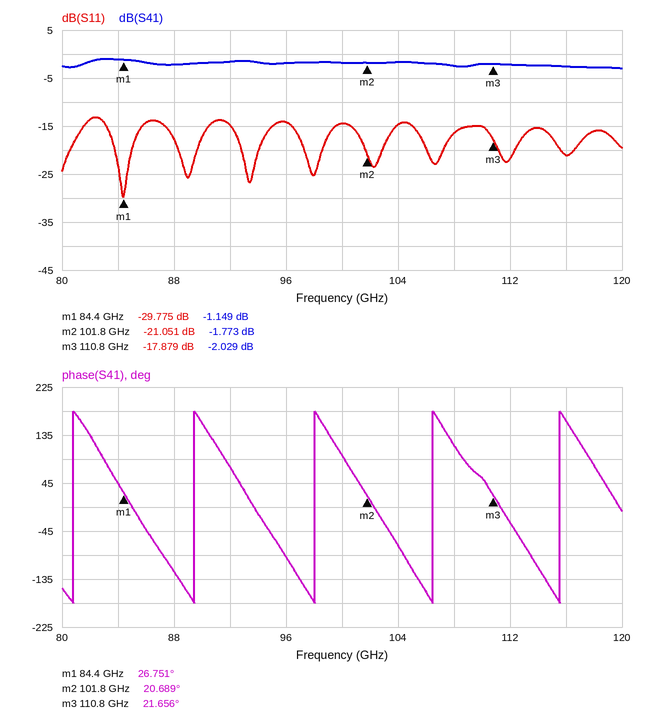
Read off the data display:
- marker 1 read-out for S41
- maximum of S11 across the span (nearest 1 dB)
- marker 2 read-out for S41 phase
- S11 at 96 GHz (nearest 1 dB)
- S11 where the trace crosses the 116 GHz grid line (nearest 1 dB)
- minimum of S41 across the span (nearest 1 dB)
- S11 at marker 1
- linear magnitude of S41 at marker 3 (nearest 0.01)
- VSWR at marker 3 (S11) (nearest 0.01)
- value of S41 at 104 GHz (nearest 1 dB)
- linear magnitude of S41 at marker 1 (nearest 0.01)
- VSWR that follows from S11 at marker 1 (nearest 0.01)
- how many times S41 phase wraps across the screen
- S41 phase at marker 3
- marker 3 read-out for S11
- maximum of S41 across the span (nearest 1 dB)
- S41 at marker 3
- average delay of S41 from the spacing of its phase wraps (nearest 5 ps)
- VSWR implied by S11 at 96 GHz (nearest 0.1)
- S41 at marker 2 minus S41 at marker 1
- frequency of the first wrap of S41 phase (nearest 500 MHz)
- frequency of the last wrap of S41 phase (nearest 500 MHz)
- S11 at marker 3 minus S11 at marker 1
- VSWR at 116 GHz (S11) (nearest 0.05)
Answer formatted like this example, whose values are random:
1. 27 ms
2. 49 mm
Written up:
1. -1.149 dB
2. -13 dB
3. 20.689°
4. -14 dB
5. -21 dB
6. -3 dB
7. -29.775 dB
8. 0.79
9. 1.29
10. -2 dB
11. 0.88
12. 1.07
13. 5
14. 21.656°
15. -17.879 dB
16. -1 dB
17. -2.029 dB
18. 115 ps
19. 1.5
20. -0.624 dB
21. 81.0 GHz
22. 115.5 GHz
23. 11.896 dB
24. 1.20
